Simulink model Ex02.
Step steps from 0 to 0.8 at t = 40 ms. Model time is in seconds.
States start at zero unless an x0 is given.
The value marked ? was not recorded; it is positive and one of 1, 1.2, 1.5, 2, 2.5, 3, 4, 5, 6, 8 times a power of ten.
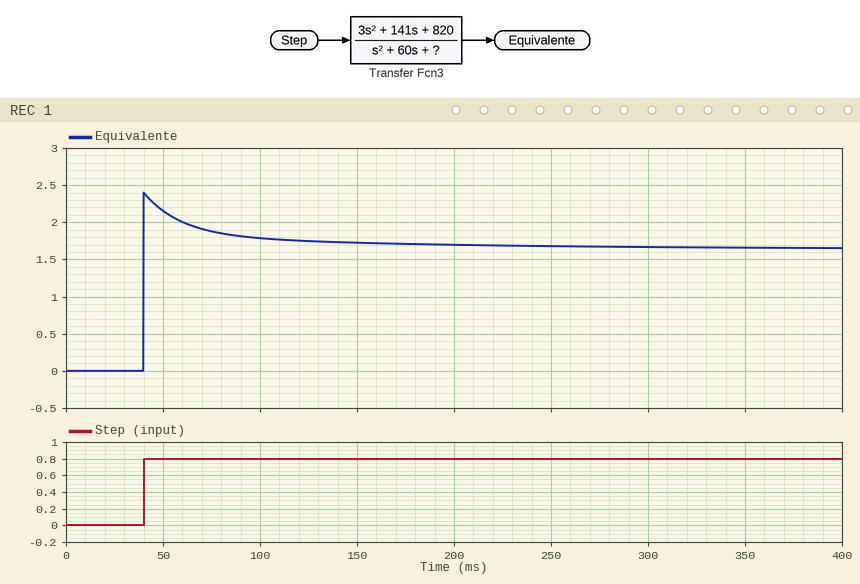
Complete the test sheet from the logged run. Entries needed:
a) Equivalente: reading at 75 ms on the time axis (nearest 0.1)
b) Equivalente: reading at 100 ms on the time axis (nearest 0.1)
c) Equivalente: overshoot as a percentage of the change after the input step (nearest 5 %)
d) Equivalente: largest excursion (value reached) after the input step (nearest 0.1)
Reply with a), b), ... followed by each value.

a) 1.9
b) 1.8
c) 45 %
d) 2.4
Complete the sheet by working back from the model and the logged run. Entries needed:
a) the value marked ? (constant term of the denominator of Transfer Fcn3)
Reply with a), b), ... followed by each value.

a) 400
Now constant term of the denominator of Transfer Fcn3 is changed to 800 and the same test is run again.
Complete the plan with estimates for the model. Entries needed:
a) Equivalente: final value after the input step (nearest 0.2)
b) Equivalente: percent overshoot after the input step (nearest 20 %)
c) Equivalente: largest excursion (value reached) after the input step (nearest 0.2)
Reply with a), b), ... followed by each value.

a) 0.8
b) 200 %
c) 2.4
